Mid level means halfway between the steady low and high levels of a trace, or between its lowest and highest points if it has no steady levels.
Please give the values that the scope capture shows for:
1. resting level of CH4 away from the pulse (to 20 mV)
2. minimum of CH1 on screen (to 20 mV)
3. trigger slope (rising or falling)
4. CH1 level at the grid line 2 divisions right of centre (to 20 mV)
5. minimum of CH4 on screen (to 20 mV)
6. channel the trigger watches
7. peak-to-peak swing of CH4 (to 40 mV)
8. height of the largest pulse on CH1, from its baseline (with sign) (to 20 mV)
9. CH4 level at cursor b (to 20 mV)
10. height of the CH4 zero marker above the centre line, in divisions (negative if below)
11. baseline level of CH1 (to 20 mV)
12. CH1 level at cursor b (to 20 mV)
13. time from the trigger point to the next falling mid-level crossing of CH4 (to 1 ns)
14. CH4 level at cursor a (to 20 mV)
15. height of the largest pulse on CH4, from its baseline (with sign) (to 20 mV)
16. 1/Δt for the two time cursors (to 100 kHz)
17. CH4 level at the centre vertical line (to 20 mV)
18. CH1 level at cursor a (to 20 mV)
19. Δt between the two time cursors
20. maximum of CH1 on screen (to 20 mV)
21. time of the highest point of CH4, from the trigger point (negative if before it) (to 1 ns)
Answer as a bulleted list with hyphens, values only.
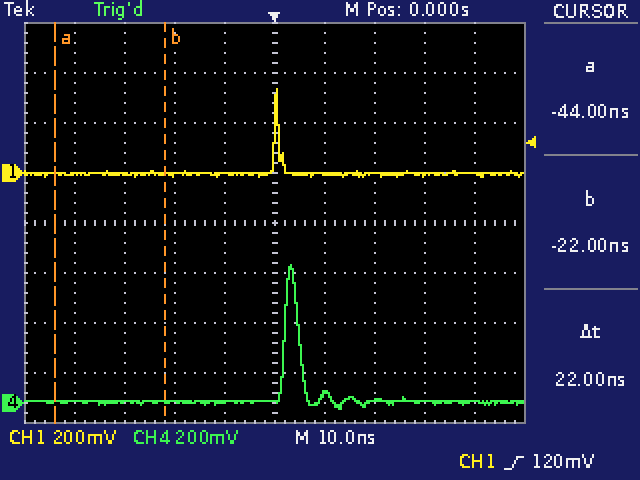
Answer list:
- 0 mV
- -20 mV
- rising
- 0 mV
- -20 mV
- CH1
- 560 mV
- +340 mV
- 0 mV
- -3.6 div
- 0 mV
- 0 mV
- 5 ns
- 0 mV
- +540 mV
- 45.5 MHz
- 0 mV
- 0 mV
- 22 ns
- 340 mV
- +3 ns
